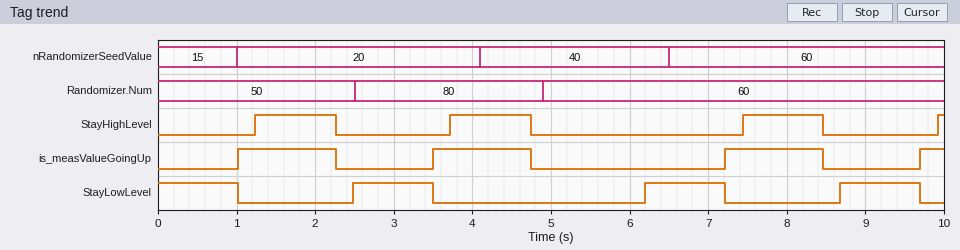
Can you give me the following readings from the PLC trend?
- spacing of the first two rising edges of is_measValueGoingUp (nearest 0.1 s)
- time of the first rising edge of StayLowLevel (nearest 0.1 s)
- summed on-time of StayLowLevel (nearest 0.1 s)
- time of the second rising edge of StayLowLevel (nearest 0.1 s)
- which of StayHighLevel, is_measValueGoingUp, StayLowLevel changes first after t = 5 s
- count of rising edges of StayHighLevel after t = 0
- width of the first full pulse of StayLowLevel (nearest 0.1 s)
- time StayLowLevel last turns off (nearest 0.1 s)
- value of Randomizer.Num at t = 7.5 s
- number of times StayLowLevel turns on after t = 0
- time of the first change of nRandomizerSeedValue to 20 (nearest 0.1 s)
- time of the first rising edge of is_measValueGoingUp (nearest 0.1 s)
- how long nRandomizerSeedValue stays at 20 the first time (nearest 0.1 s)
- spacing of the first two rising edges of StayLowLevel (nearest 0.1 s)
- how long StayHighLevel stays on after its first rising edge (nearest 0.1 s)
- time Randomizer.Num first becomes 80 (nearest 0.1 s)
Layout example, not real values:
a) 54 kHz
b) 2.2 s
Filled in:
a) 2.5 s
b) 2.5 s
c) 4.1 s
d) 6.2 s
e) StayLowLevel
f) 4
g) 1.0 s
h) 9.7 s
i) 60
j) 3
k) 1.0 s
l) 1.0 s
m) 3.1 s
n) 3.7 s
o) 1.0 s
p) 2.5 s
